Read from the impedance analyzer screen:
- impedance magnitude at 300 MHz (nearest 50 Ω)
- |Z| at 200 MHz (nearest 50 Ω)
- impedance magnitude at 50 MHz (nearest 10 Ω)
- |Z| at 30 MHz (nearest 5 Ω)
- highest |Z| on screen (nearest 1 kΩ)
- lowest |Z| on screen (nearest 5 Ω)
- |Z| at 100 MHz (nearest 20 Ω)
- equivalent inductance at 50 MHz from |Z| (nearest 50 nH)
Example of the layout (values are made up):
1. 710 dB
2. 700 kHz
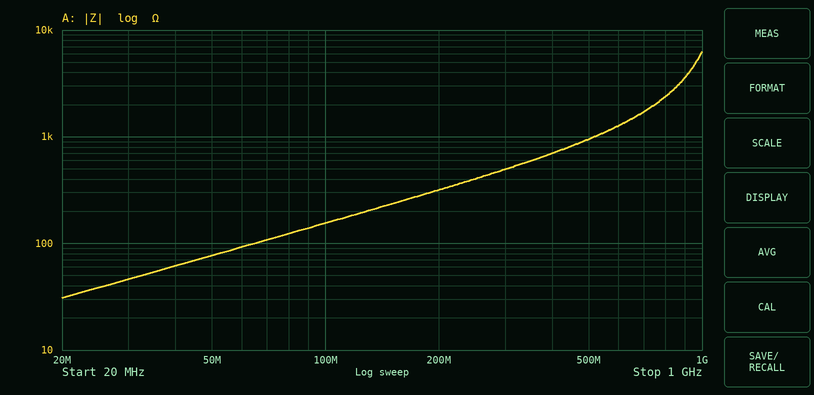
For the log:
1. 500 Ω
2. 300 Ω
3. 80 Ω
4. 45 Ω
5. 6 kΩ
6. 30 Ω
7. 160 Ω
8. 250 nH
